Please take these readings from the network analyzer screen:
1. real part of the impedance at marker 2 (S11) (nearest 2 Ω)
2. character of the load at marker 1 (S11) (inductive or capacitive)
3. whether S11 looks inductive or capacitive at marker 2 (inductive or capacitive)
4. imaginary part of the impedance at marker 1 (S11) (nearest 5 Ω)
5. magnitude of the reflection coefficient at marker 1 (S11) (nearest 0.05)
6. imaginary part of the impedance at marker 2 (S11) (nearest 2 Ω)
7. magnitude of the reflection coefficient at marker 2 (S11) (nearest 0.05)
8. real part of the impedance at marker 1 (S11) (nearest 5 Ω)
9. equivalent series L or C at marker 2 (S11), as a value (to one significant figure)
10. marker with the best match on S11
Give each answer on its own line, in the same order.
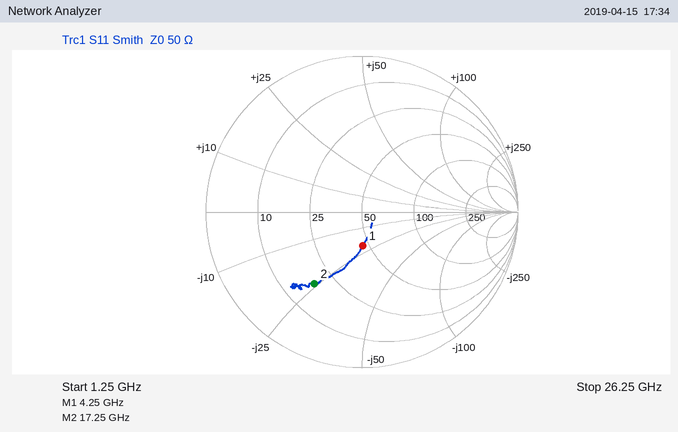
18 Ω
capacitive
capacitive
-20 Ω
0.20
-24 Ω
0.55
45 Ω
400 fF
marker 1
